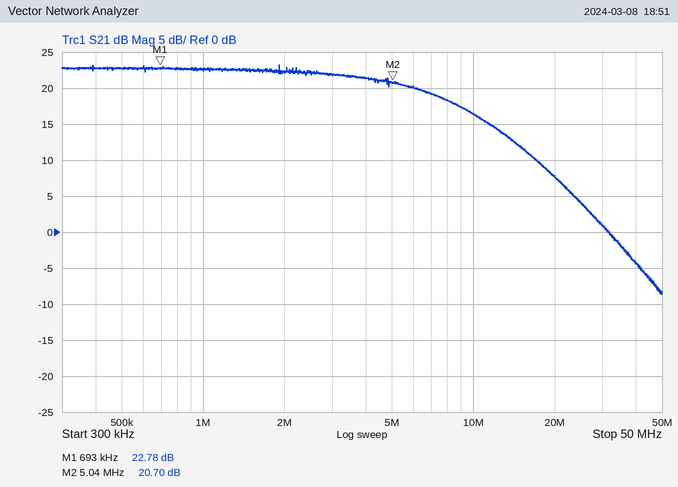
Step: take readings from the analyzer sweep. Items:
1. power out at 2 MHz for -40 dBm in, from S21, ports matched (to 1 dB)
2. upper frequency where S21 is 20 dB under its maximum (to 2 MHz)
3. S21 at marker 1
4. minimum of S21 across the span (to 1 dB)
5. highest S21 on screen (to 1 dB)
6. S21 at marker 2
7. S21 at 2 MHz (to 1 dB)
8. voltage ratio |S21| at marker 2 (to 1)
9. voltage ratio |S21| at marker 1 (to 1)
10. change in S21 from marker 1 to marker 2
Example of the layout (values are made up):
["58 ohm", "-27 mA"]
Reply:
["-18 dBm", "26 MHz", "22.78 dB", "-9 dB", "23 dB", "20.70 dB", "22 dB", "11", "14", "-2.08 dB"]
